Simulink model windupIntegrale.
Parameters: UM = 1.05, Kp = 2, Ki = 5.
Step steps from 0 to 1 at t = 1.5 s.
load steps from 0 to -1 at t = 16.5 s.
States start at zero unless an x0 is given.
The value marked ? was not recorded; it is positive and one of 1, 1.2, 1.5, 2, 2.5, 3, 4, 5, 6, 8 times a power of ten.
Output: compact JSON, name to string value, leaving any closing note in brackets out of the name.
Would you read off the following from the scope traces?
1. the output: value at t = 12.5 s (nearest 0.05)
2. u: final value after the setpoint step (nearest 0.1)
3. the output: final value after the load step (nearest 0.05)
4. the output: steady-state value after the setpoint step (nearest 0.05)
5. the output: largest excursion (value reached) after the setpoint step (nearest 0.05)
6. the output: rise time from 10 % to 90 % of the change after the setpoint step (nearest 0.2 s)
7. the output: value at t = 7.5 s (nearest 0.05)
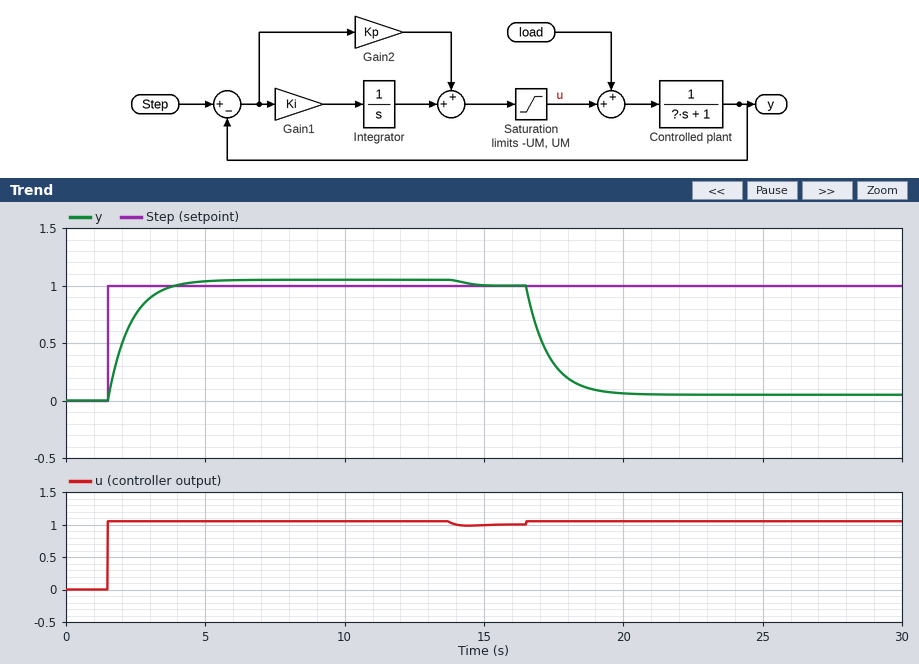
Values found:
{"the output: value at t = 12.5 s": "1.05", "u: final value after the setpoint step": "1.0", "the output: final value after the load step": "0.05", "the output: steady-state value after the setpoint step": "1.00", "the output: largest excursion (value reached) after the setpoint step": "1.05", "the output: rise time from 10 % to 90 % of the change after the setpoint step": "1.4 s", "the output: value at t = 7.5 s": "1.05"}
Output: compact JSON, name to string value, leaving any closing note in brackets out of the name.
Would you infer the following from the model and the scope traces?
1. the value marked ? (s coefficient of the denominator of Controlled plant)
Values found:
{"the value marked ?": "0.8"}
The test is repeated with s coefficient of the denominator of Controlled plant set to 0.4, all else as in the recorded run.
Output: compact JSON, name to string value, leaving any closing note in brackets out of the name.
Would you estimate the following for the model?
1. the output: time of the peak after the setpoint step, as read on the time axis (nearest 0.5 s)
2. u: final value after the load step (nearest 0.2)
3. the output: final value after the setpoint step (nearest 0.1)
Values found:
{"the output: time of the peak after the setpoint step, as read on the time axis": "5.5 s", "u: final value after the load step": "1.0", "the output: final value after the setpoint step": "1.0"}
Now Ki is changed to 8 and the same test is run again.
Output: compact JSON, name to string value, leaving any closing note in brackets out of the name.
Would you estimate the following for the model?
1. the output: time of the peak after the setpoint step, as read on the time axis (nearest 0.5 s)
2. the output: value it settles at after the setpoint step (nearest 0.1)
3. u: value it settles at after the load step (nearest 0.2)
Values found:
{"the output: time of the peak after the setpoint step, as read on the time axis": "15.5 s", "the output: value it settles at after the setpoint step": "1.0", "u: value it settles at after the load step": "1.0"}
